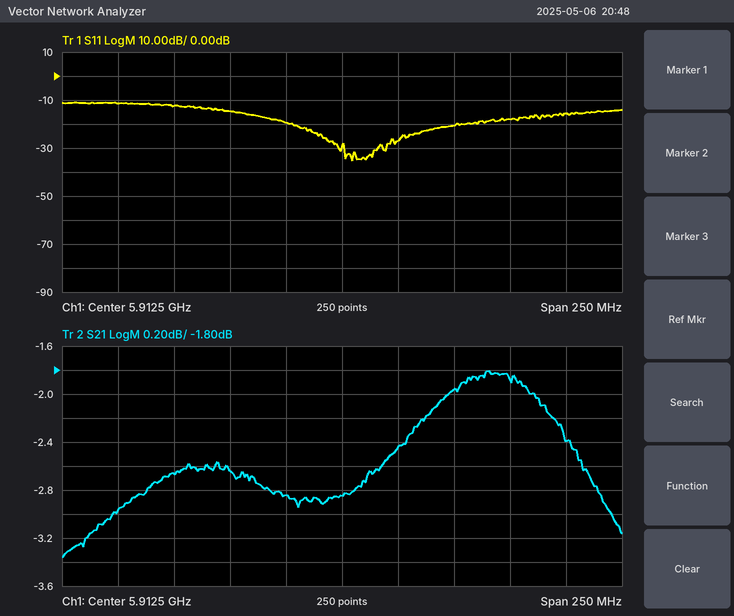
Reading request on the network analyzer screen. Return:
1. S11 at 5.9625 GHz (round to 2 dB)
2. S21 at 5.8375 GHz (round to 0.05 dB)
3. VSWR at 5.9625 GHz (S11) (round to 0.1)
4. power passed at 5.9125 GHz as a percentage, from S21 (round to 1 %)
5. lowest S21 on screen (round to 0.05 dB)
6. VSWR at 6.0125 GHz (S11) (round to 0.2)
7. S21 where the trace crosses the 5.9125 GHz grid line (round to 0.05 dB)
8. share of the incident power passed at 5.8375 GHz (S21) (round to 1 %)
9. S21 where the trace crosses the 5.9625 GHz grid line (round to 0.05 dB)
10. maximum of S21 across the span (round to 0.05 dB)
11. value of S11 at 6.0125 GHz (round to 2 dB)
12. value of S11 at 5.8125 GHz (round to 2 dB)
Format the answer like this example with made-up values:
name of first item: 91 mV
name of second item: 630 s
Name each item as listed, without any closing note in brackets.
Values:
S11 at 5.9625 GHz: -20 dB
S21 at 5.8375 GHz: -2.65 dB
VSWR at 5.9625 GHz (S11): 1.2
power passed at 5.9125 GHz as a percentage, from S21: 52 %
lowest S21 on screen: -3.35 dB
VSWR at 6.0125 GHz (S11): 1.4
S21 where the trace crosses the 5.9125 GHz grid line: -2.85 dB
share of the incident power passed at 5.8375 GHz (S21): 54 %
S21 where the trace crosses the 5.9625 GHz grid line: -1.95 dB
maximum of S21 across the span: -1.80 dB
value of S11 at 6.0125 GHz: -16 dB
value of S11 at 5.8125 GHz: -12 dB
